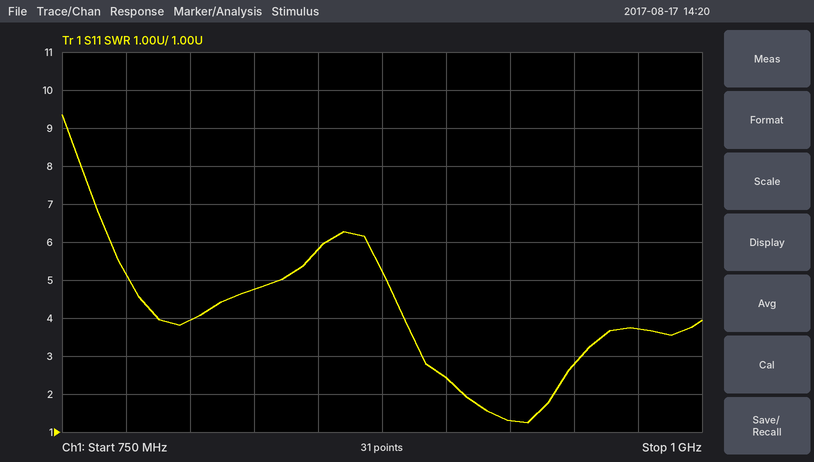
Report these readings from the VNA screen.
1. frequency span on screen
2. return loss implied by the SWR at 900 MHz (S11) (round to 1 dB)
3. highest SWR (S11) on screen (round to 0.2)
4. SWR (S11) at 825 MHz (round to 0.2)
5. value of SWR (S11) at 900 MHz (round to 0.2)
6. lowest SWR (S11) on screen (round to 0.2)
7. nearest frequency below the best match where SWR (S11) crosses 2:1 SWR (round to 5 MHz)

250 MHz
8 dB
9.4
4.8
2.4
1.2
905 MHz
